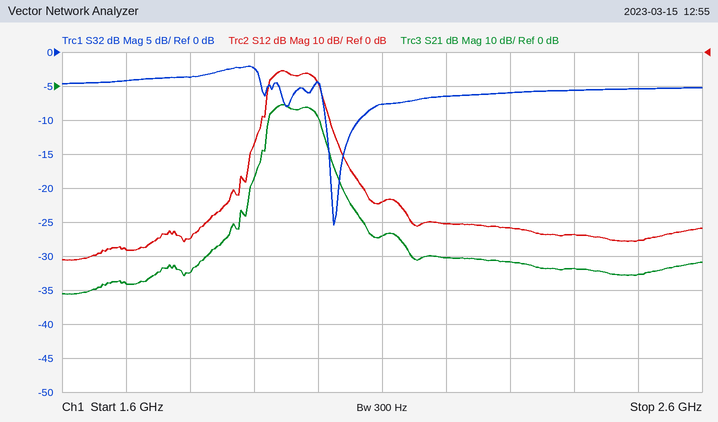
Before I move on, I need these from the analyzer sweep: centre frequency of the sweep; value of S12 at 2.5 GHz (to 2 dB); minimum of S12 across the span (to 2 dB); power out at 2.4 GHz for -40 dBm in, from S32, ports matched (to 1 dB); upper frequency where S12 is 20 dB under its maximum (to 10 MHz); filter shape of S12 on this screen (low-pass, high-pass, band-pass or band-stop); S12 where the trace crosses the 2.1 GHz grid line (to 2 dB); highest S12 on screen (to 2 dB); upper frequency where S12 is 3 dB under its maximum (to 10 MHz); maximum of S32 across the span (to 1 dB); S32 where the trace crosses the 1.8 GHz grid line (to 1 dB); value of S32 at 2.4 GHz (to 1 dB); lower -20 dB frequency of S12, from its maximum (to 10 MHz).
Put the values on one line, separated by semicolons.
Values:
2.1 GHz; -56 dB; -62 dB; -46 dBm; 2.03 GHz; band-pass; -44 dB; -6 dB; 2.00 GHz; -2 dB; -4 dB; -6 dB; 1.90 GHz
